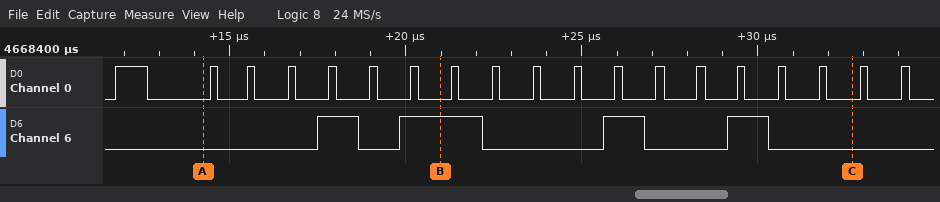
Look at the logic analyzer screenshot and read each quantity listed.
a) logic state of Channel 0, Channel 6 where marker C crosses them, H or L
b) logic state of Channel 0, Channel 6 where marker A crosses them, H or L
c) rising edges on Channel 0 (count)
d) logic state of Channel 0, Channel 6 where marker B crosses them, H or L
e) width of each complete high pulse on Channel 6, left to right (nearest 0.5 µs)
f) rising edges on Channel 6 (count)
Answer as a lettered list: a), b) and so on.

a) Channel 0=L, Channel 6=L
b) Channel 0=L, Channel 6=L
c) 19
d) Channel 0=L, Channel 6=H
e) 1 µs, 2.5 µs, 1 µs, 1 µs
f) 4
